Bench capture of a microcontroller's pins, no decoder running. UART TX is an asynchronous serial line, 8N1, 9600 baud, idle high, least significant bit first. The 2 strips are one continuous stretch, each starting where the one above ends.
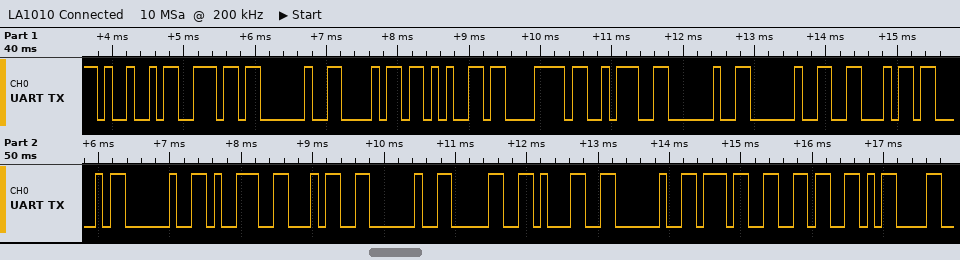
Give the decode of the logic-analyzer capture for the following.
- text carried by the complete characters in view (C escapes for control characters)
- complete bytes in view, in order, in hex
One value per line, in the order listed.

"In hex:  FC 94 01 76\r"
49 6E 20 68 65 78 3A 20 20 46 43 20 39 34 20 30 31 20 37 36 0D
